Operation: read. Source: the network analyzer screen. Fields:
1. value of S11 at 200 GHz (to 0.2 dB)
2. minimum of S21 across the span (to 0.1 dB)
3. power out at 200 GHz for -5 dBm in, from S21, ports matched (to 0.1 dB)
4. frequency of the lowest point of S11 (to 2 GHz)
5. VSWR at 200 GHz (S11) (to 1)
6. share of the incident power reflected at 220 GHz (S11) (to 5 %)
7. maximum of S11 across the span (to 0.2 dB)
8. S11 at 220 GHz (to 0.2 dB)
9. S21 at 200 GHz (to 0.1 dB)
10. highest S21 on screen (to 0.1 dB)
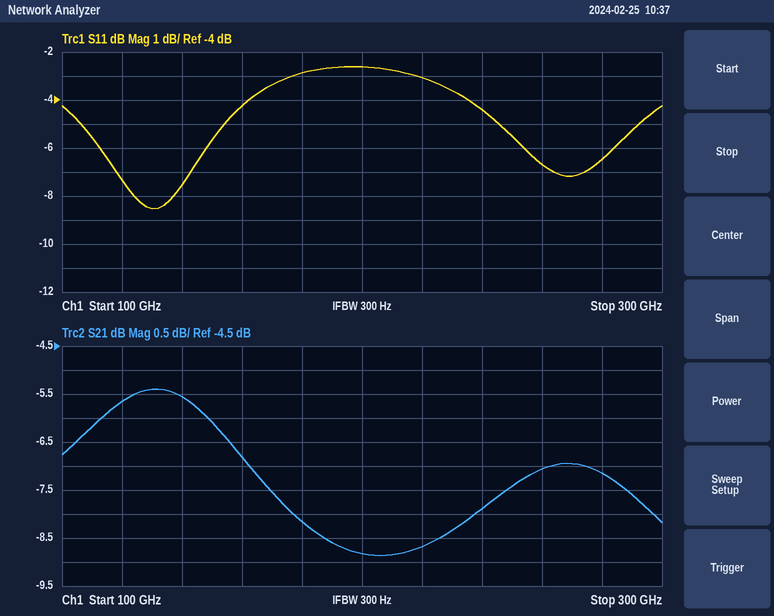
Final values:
-2.6 dB
-8.9 dB
-13.8 dBm
130 GHz
7
50 %
-2.6 dB
-3.0 dB
-8.8 dB
-5.4 dB
